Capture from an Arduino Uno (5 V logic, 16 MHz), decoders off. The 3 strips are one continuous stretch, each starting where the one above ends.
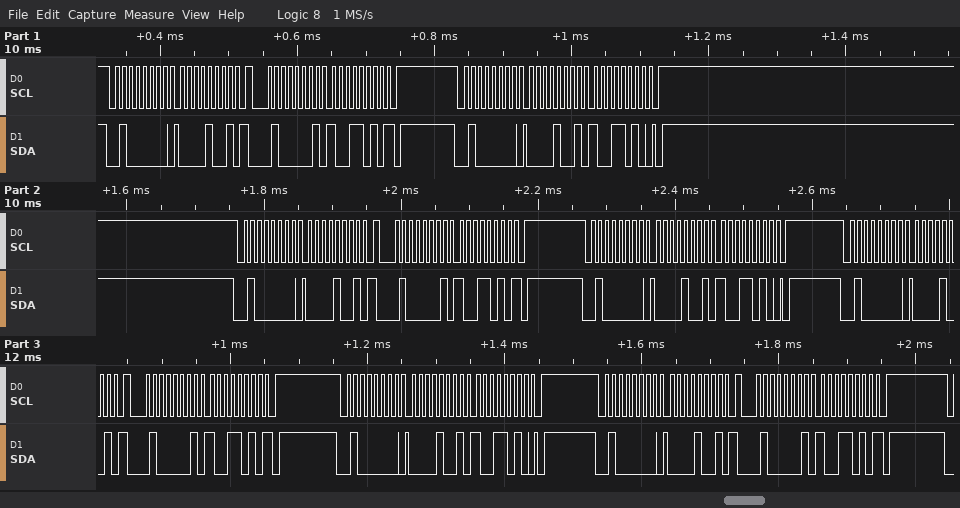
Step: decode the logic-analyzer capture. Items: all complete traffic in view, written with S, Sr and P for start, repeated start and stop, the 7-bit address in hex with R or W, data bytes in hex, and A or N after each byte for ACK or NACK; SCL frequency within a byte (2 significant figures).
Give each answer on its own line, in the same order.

S 20W A 09 A Sr 20R A 9A N P S 20W A 09 A 9A A P S 20W A 09 A Sr 20R A 9A N P S 20W A 09 A 9A A P S 20W A 09 A Sr 20R A 9A N P S 20W A 09 A 9A A P S 20W A 09 A Sr 20R A 9A N P
100 kHz
